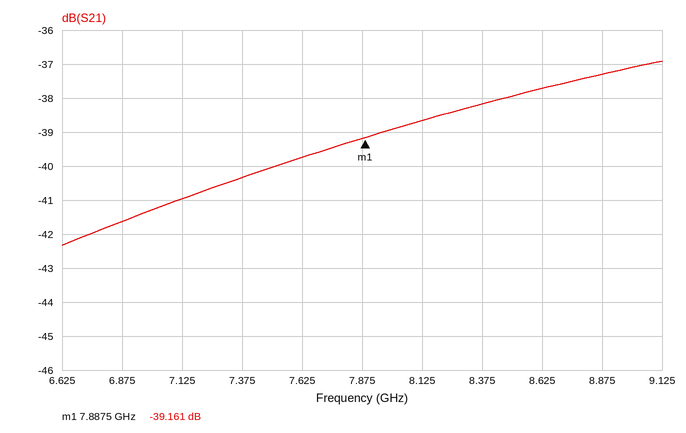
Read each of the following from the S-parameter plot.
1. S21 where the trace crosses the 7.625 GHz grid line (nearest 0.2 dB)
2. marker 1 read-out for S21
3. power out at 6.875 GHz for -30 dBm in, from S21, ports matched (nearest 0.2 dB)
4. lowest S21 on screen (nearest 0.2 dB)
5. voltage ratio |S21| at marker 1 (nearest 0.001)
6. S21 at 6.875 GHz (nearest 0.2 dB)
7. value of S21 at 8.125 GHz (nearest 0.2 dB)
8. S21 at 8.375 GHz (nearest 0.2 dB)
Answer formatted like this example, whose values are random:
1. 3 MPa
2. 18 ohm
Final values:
1. -39.8 dB
2. -39.161 dB
3. -71.6 dBm
4. -42.4 dB
5. 0.011
6. -41.6 dB
7. -38.6 dB
8. -38.2 dB
